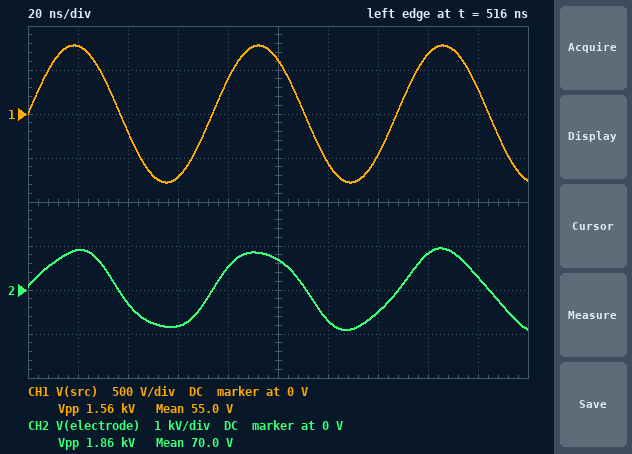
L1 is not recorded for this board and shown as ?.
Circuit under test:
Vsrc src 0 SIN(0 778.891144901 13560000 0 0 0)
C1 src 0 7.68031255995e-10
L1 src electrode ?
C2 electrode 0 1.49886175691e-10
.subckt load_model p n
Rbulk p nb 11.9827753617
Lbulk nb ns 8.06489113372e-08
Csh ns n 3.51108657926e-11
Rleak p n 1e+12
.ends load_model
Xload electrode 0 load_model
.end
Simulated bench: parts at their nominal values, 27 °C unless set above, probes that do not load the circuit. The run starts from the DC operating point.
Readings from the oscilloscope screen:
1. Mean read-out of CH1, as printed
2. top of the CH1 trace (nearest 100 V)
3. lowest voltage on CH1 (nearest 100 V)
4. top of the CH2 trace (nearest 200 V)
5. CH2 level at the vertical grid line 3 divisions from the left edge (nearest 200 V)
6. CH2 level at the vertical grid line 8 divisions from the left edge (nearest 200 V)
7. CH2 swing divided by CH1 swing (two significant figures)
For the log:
55.0 V
800 V
-800 V
1.0 kV
-800 V
800 V
1.2
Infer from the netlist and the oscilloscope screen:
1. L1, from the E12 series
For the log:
100 nH
